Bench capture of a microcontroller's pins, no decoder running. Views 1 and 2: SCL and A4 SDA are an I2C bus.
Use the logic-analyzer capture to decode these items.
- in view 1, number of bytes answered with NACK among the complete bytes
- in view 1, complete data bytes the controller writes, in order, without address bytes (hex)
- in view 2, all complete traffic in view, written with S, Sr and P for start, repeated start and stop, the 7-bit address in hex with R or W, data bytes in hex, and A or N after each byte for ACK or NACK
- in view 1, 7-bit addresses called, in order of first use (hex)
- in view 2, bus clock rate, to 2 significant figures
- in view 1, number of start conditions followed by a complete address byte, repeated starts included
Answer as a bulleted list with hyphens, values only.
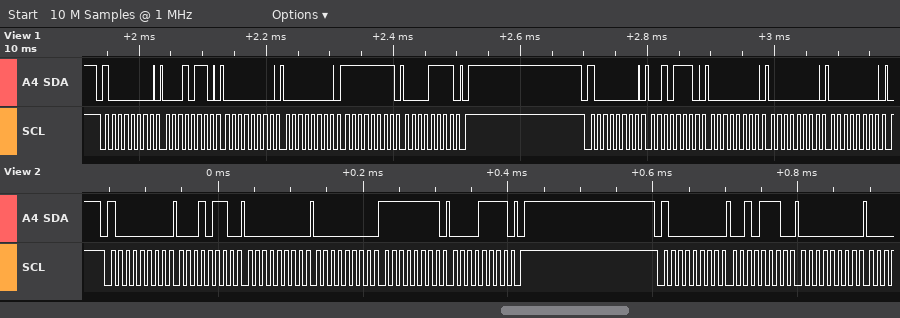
- 0
- 16 00 00 FF 0F 2E 00 00 00
- S 40W A 16 A 00 A 00 A FF A 0F A P S 40W A 2E A 00 A
- 0x40
- 100 kHz
- 2
